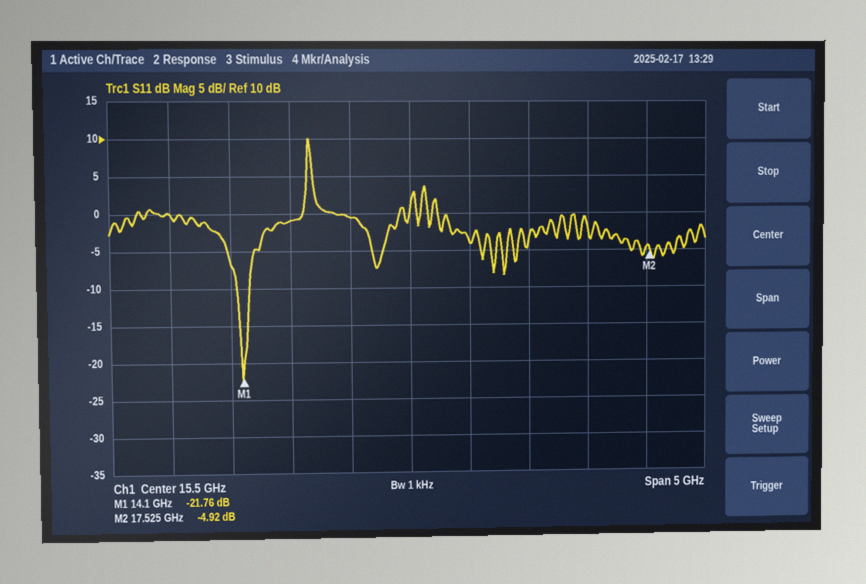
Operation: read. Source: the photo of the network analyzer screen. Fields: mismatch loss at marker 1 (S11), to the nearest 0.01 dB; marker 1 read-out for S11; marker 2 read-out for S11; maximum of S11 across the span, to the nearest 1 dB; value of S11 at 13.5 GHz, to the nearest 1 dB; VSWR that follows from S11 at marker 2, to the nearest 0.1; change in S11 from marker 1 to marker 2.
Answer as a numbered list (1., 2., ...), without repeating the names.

1. 0.03 dB
2. -21.76 dB
3. -4.92 dB
4. 10 dB
5. 0 dB
6. 3.6
7. 16.84 dB
